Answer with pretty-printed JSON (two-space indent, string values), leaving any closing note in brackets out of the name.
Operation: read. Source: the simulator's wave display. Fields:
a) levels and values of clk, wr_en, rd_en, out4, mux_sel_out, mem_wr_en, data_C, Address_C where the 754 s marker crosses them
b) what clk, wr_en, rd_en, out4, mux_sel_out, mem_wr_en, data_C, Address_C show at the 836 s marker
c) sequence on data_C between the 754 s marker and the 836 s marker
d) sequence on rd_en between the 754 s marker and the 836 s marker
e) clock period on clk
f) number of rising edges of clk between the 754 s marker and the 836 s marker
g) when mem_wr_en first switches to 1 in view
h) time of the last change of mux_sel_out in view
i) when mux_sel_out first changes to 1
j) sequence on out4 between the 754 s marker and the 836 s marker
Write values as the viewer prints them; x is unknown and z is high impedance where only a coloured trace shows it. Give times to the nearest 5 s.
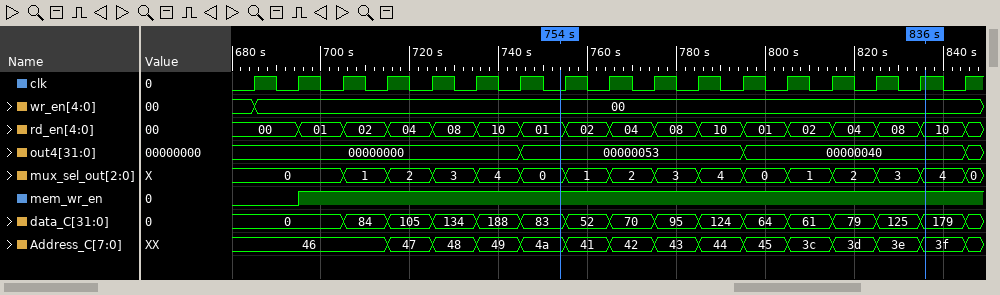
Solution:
{
  "levels and values of clk, wr_en, rd_en, out4, mux_sel_out, mem_wr_en, data_C, Address_C where the 754 s marker crosses them": "clk=0, wr_en=00, rd_en=01, out4=00000053, mux_sel_out=0, mem_wr_en=1, data_C=83, Address_C=4a",
  "what clk, wr_en, rd_en, out4, mux_sel_out, mem_wr_en, data_C, Address_C show at the 836 s marker": "clk=1, wr_en=00, rd_en=10, out4=00000040, mux_sel_out=4, mem_wr_en=1, data_C=179, Address_C=3f",
  "sequence on data_C between the 754 s marker and the 836 s marker": "83, 52, 70, 95, 124, 64, 61, 79, 125, 179",
  "sequence on rd_en between the 754 s marker and the 836 s marker": "01, 02, 04, 08, 10, 01, 02, 04, 08, 10",
  "clock period on clk": "10 s",
  "number of rising edges of clk between the 754 s marker and the 836 s marker": "9",
  "when mem_wr_en first switches to 1 in view": "695 s",
  "time of the last change of mux_sel_out in view": "845 s",
  "when mux_sel_out first changes to 1": "705 s",
  "sequence on out4 between the 754 s marker and the 836 s marker": "00000053, 00000040"
}
